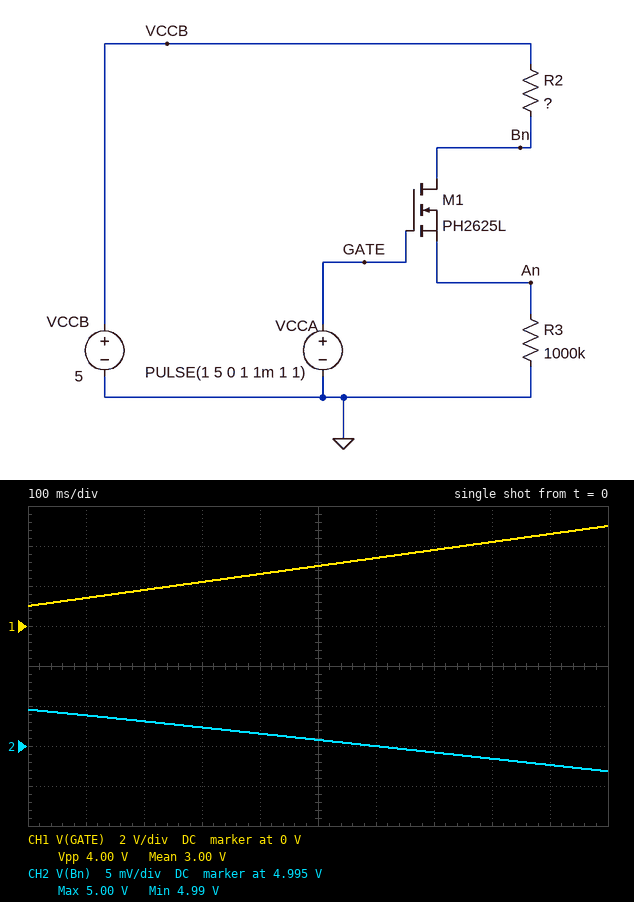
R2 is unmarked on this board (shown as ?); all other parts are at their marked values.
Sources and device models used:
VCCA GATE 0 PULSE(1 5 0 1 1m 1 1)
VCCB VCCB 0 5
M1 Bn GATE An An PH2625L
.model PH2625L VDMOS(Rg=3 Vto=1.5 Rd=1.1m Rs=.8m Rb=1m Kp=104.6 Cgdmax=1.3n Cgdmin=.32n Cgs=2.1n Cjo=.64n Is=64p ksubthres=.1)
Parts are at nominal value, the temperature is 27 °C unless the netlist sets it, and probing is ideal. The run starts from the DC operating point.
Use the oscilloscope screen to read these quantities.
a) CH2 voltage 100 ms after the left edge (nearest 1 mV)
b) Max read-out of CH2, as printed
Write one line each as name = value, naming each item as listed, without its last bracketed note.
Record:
CH2 voltage 100 ms after the left edge = 4.999 V
Max read-out of CH2, as printed = 5.00 V
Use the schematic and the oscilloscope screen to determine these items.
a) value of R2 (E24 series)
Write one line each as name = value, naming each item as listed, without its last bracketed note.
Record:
value of R2 = 2 kΩ
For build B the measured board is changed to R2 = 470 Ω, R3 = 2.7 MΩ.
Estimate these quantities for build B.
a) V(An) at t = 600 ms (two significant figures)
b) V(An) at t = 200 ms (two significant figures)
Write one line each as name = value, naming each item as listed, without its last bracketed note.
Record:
V(An) at t = 600 ms = 2.6 V
V(An) at t = 200 ms = 1.0 V
